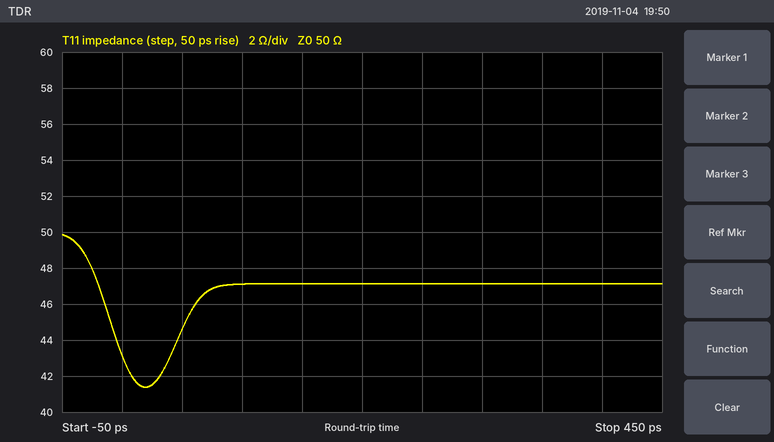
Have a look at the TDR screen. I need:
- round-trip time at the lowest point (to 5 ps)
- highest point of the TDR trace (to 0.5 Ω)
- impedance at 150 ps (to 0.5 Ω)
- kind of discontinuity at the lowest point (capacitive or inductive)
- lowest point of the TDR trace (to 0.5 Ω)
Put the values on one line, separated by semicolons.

20 ps; 50.0 Ω; 47.0 Ω; capacitive; 41.5 Ω
